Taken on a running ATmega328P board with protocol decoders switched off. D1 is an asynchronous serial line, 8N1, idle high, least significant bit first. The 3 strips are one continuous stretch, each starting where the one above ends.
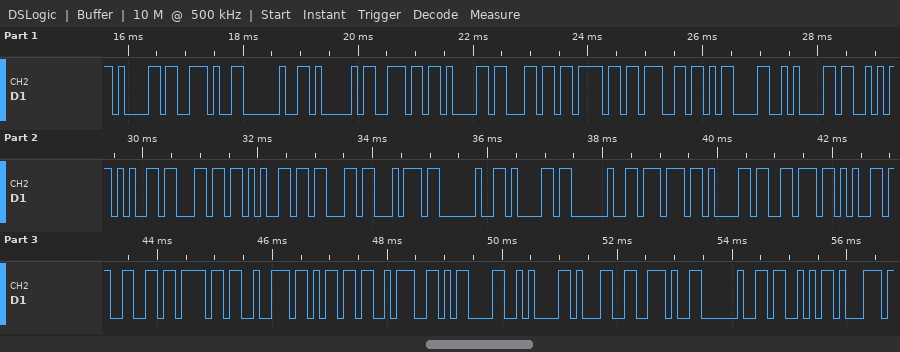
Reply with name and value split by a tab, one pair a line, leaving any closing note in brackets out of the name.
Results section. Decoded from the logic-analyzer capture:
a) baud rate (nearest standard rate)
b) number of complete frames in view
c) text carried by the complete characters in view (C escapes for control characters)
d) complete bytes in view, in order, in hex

baud rate	9600 baud
number of complete frames in view	36
text carried by the complete characters in view	"a. Analog\r\nSelect a waveform:\r\n1. Sq"
complete bytes in view, in order, in hex	61 2E 20 41 6E 61 6C 6F 67 0D 0A 53 65 6C 65 63 74 20 61 20 77 61 76 65 66 6F 72 6D 3A 0D 0A 31 2E 20 53 71
